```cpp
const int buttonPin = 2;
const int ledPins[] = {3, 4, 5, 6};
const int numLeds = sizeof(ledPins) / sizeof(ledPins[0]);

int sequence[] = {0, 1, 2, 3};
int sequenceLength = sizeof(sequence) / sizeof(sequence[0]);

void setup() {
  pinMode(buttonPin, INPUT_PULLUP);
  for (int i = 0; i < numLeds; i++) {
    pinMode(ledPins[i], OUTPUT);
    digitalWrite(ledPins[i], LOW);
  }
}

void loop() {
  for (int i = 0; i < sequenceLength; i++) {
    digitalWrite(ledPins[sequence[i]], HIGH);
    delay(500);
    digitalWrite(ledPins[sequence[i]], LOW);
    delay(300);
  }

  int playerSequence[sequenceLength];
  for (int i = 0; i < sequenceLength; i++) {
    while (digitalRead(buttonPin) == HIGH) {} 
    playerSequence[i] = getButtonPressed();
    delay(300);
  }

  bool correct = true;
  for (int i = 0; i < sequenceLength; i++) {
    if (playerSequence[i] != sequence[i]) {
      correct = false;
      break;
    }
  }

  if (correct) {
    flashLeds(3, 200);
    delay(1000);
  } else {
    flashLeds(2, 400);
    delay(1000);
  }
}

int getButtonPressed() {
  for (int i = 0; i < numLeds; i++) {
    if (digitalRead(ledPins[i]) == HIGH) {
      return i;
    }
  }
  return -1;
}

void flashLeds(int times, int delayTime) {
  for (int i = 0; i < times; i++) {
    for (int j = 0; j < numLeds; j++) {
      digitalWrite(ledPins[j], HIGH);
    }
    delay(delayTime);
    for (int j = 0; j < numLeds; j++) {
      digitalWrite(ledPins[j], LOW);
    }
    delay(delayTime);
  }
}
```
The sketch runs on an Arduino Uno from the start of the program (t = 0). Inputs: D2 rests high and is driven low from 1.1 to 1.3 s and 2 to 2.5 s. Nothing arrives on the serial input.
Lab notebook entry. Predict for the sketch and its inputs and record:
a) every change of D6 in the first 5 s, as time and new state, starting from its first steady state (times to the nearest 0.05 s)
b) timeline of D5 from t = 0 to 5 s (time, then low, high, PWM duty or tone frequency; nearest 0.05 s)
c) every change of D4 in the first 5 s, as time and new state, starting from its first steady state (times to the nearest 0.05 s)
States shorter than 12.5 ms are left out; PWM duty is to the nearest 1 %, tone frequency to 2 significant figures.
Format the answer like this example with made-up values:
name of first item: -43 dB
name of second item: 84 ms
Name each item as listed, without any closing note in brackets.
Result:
every change of D6 in the first 5 s, as time and new state, starting from its first steady state: 0 s low; 2.4 s high; 2.9 s low
timeline of D5 from t = 0 to 5 s: 0 s low; 1.6 s high; 2.1 s low
every change of D4 in the first 5 s, as time and new state, starting from its first steady state: 0 s low; 0.8 s high; 1.3 s low
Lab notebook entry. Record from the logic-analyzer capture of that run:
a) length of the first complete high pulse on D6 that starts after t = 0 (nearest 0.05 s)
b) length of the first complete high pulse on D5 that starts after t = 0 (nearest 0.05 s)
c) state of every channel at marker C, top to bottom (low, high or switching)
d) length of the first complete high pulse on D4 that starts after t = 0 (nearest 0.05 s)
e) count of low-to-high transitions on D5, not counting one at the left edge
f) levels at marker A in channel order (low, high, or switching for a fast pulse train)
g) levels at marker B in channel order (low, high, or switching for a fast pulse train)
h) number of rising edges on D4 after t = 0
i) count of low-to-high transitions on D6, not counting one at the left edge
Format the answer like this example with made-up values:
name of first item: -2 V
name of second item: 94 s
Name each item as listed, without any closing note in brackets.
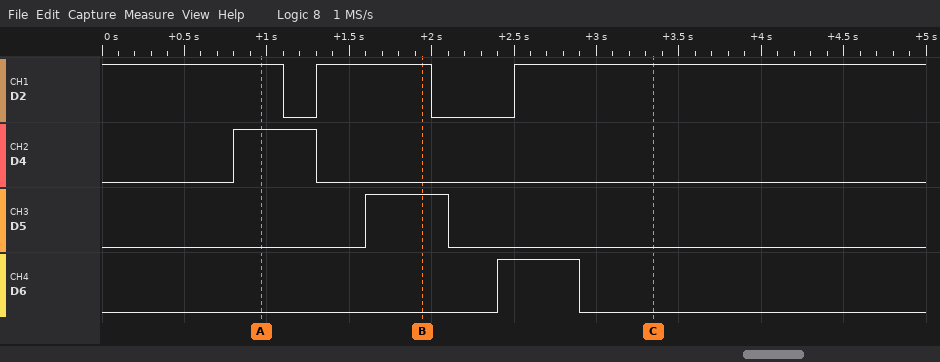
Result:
length of the first complete high pulse on D6 that starts after t = 0: 0.50 s
length of the first complete high pulse on D5 that starts after t = 0: 0.50 s
state of every channel at marker C, top to bottom: D2 high, D4 low, D5 low, D6 low
length of the first complete high pulse on D4 that starts after t = 0: 0.50 s
count of low-to-high transitions on D5, not counting one at the left edge: 1
levels at marker A in channel order: D2 high, D4 high, D5 low, D6 low
levels at marker B in channel order: D2 high, D4 low, D5 high, D6 low
number of rising edges on D4 after t = 0: 1
count of low-to-high transitions on D6, not counting one at the left edge: 1
